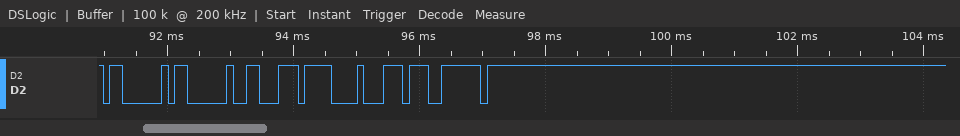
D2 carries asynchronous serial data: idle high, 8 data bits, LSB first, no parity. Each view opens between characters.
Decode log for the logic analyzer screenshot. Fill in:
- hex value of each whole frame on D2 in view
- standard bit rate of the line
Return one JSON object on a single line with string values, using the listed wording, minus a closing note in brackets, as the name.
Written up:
{"hex value of each whole frame on D2 in view": "03, 03, C6, 0F, DC, 7E", "standard bit rate of the line": "9600 baud"}
